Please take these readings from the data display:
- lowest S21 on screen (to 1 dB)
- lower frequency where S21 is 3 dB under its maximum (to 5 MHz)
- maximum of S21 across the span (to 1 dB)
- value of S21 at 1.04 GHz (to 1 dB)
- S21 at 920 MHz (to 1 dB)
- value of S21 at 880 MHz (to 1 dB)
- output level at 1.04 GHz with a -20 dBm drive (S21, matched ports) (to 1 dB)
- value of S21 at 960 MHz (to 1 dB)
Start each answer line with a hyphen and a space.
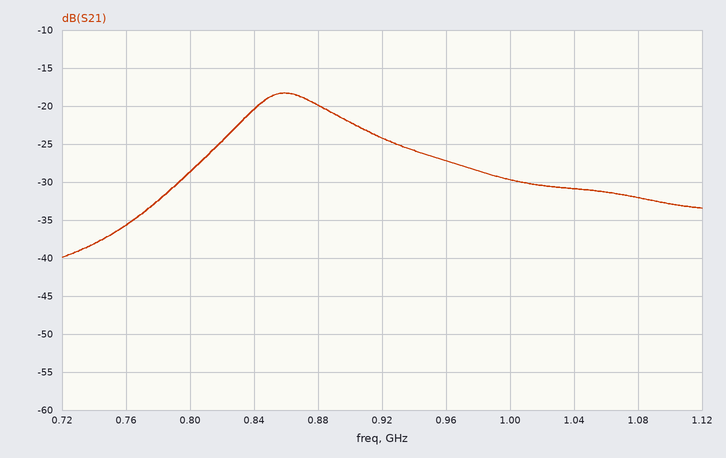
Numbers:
- -40 dB
- 835 MHz
- -18 dB
- -31 dB
- -24 dB
- -20 dB
- -51 dBm
- -27 dB
